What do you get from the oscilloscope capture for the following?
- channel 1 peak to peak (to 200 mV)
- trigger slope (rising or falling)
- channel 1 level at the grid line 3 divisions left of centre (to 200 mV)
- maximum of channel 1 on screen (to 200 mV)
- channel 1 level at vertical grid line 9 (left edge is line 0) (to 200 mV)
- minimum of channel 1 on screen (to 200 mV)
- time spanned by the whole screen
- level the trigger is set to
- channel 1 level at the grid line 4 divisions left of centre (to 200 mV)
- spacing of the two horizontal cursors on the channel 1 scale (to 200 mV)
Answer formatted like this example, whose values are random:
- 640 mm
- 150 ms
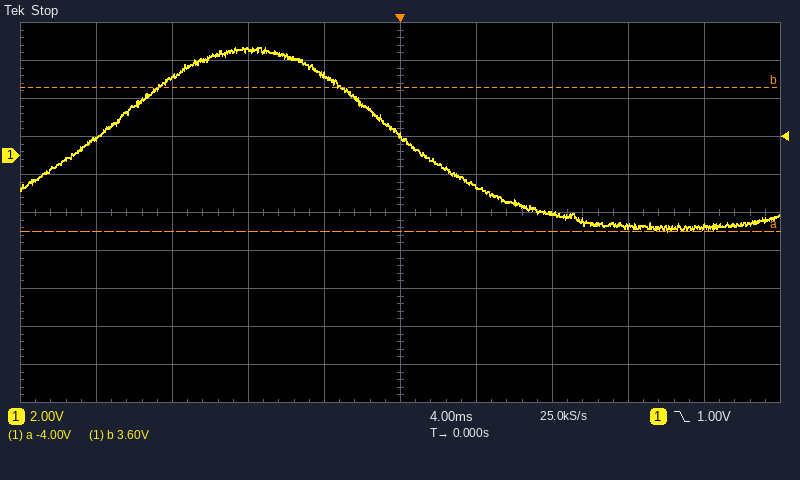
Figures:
- 9.6 V
- falling
- 4.2 V
- 5.6 V
- -3.8 V
- -4.0 V
- 40 ms
- 1.00 V
- 1.0 V
- 7.6 V
